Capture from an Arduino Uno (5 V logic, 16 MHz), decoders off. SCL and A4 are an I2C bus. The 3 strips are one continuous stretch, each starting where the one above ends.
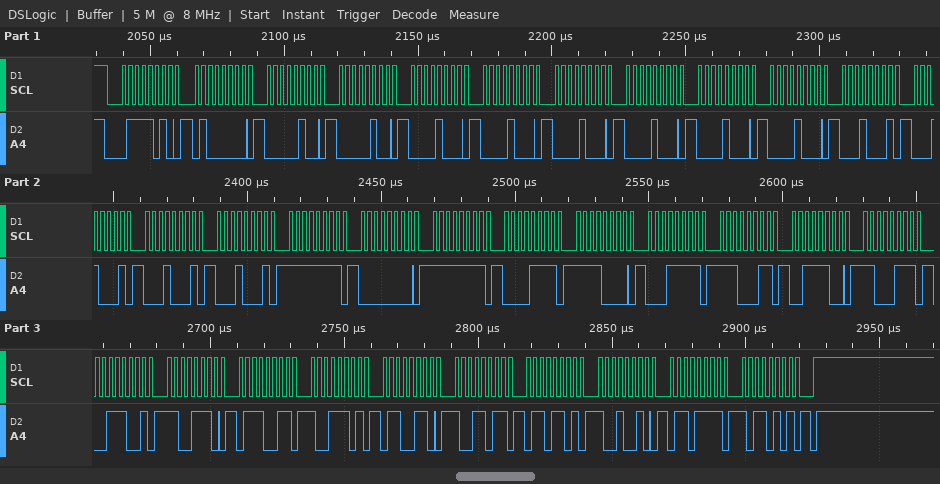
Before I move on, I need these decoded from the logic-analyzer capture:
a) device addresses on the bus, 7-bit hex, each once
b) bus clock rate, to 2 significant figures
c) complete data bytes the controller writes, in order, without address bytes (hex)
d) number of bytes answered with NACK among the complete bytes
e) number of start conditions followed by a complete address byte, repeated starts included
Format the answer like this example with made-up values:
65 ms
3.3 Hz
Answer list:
0x3D
400 kHz
40 04 04 08 08 08 08 08 08 11 11 11 11 FF 00 FF 0F F0 1F E3 3C C7 39 CE 73 9D 66 9B 6D 92 6F B5
0
1
